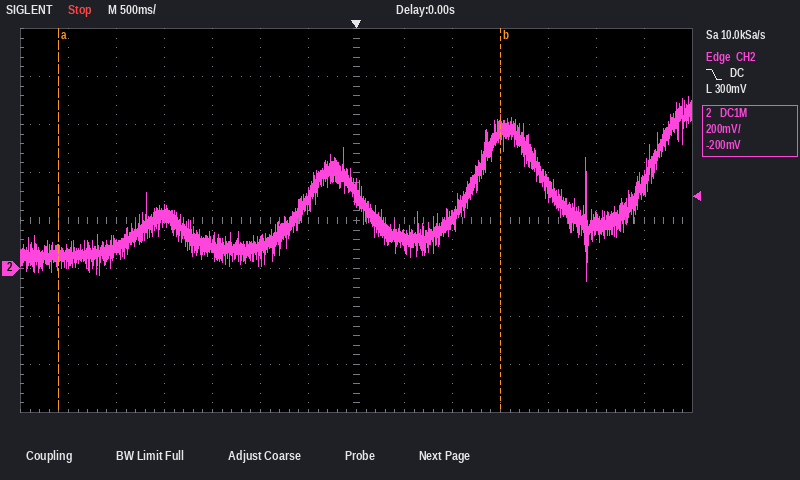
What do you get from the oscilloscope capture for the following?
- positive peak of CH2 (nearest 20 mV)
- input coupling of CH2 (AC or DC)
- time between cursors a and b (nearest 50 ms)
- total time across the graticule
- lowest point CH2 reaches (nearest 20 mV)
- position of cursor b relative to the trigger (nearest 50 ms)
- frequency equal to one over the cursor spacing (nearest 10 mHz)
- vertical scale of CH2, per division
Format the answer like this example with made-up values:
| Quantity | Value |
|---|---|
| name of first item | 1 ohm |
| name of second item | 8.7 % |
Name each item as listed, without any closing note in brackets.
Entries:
| Quantity | Value |
|---|---|
| positive peak of CH2 | 720 mV |
| input coupling of CH2 | DC |
| time between cursors a and b | 4.60 s |
| total time across the graticule | 7 s |
| lowest point CH2 reaches | -60 mV |
| position of cursor b relative to the trigger | +1.50 s |
| frequency equal to one over the cursor spacing | 220 mHz |
| vertical scale of CH2, per division | 200 mV |
